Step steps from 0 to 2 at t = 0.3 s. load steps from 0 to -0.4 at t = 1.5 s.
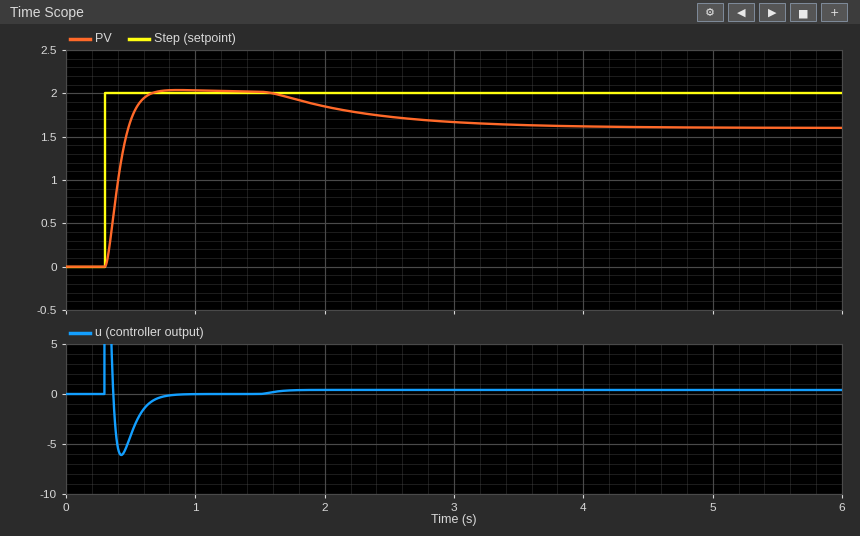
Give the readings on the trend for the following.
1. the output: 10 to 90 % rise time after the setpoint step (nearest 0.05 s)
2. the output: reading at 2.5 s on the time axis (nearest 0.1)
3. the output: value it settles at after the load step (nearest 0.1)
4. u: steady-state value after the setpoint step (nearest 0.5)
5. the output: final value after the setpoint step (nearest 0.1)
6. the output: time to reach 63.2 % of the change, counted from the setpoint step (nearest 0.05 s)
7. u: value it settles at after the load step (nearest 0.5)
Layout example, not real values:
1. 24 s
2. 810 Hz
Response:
1. 0.20 s
2. 1.7
3. 1.6
4. 0.0
5. 2.0
6. 0.15 s
7. 0.5
